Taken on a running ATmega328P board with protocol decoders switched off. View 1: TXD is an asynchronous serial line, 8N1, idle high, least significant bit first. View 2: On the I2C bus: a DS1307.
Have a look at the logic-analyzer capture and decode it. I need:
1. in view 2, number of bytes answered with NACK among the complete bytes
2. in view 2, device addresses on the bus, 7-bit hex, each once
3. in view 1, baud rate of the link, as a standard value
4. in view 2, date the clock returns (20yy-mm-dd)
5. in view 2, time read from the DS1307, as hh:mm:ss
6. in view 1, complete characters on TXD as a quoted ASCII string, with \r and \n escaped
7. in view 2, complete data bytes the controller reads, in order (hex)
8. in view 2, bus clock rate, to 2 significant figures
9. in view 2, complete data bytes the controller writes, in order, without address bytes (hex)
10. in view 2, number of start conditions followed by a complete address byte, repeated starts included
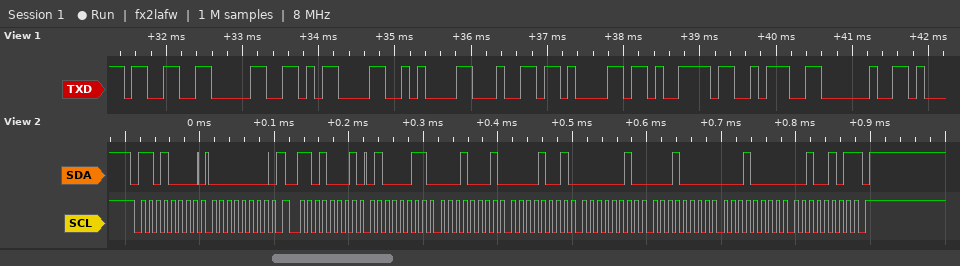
1
0x68
9600 baud
2025-10-10
09:11:43
"30\r\nday: "
43 11 09 02 10 10 25
100 kHz
00
2
